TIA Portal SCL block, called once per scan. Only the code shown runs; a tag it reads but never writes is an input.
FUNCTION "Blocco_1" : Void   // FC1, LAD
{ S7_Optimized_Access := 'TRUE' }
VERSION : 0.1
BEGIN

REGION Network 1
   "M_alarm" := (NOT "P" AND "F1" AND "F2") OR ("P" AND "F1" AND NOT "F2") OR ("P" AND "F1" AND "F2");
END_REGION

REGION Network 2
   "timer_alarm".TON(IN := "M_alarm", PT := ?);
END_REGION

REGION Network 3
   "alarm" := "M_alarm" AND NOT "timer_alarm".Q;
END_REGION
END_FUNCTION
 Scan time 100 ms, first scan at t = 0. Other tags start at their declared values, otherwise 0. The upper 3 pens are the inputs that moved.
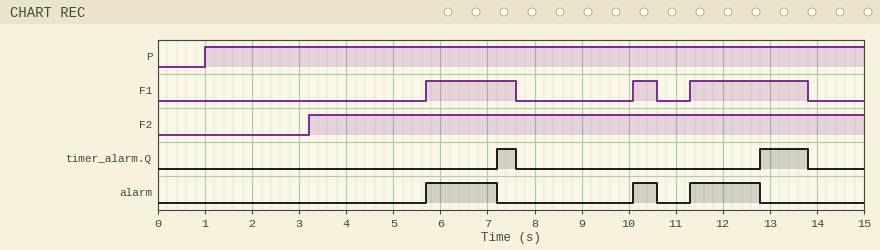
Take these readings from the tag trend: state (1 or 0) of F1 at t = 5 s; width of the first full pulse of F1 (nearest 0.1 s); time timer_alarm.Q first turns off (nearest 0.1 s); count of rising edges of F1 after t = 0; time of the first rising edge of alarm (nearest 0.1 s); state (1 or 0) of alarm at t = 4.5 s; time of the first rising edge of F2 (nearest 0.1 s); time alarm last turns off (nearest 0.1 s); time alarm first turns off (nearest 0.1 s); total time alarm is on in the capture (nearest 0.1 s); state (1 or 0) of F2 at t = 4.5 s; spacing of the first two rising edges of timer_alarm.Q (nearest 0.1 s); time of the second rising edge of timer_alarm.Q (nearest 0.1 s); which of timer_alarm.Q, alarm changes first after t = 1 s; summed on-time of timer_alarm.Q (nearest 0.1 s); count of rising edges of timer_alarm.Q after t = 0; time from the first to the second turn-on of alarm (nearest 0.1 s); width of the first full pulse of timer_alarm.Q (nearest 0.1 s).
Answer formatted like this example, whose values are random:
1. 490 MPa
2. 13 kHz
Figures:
1. 0
2. 1.9 s
3. 7.6 s
4. 3
5. 5.7 s
6. 0
7. 3.2 s
8. 12.8 s
9. 7.2 s
10. 3.5 s
11. 1
12. 5.6 s
13. 12.8 s
14. alarm
15. 1.4 s
16. 2
17. 4.4 s
18. 0.4 s
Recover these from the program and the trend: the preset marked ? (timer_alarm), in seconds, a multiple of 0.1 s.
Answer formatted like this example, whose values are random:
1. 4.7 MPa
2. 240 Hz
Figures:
1. 1.5 s
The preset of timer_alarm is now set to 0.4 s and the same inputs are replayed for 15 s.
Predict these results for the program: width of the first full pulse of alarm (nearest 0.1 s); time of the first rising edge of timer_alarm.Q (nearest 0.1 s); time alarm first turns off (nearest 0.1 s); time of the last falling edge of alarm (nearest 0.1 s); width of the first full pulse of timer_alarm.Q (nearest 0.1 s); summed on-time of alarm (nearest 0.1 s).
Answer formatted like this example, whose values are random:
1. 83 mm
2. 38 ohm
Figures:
1. 0.4 s
2. 6.1 s
3. 6.1 s
4. 11.7 s
5. 1.5 s
6. 1.2 s
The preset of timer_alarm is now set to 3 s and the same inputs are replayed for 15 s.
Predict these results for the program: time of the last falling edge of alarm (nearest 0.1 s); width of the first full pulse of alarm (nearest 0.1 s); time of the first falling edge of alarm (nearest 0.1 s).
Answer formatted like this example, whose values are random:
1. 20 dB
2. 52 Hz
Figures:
1. 13.8 s
2. 1.9 s
3. 7.6 s
